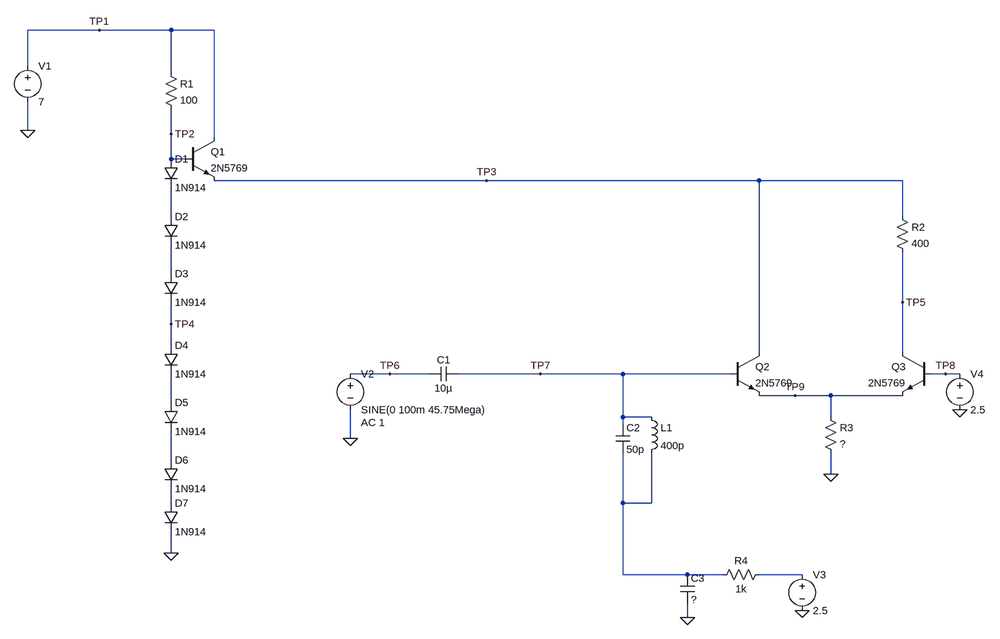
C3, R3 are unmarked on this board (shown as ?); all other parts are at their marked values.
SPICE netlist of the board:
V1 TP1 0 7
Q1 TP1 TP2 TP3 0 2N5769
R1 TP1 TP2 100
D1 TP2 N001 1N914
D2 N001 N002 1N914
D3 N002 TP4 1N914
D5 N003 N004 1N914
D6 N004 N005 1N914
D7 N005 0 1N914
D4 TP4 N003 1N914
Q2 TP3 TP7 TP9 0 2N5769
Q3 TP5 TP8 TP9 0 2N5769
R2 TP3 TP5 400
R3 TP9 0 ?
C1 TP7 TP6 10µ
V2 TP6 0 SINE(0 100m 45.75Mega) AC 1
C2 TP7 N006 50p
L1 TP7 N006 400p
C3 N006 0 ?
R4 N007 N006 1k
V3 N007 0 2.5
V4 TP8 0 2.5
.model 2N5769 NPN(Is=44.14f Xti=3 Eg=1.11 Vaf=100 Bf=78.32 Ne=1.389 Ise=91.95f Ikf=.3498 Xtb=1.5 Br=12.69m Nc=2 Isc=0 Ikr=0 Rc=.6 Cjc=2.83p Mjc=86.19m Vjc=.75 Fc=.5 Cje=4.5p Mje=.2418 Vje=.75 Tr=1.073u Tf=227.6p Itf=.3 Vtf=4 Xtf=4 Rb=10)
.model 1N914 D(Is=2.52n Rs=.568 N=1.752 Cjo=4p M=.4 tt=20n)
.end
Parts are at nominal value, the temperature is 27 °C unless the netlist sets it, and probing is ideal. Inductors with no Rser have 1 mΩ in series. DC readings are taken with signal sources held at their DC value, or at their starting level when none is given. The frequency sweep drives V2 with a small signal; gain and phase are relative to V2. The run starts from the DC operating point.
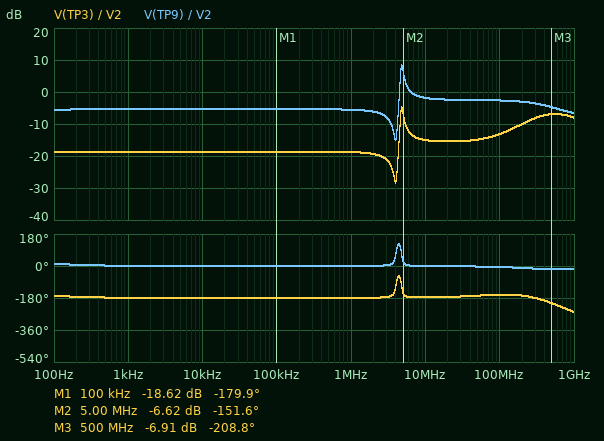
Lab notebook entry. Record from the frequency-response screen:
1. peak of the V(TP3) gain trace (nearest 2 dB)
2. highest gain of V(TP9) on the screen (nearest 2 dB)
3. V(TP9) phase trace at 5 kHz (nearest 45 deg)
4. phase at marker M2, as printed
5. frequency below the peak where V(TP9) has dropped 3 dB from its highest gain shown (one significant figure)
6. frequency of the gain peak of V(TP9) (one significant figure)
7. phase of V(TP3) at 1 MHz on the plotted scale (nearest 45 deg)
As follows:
-4 dB
8 dB
0 deg
-151.6 deg
5 MHz
5 MHz
-180 deg
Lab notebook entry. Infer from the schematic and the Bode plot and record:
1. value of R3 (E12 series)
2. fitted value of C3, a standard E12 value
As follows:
68 Ω
3.9 µF
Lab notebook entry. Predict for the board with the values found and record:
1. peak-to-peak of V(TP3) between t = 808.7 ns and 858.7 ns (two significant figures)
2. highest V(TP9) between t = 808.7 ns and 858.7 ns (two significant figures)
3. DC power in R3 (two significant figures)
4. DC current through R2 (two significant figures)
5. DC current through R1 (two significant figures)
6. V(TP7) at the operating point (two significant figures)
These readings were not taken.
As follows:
34 mV
1.8 V
43 mW
6.4 mA
19 mA
2.4 V
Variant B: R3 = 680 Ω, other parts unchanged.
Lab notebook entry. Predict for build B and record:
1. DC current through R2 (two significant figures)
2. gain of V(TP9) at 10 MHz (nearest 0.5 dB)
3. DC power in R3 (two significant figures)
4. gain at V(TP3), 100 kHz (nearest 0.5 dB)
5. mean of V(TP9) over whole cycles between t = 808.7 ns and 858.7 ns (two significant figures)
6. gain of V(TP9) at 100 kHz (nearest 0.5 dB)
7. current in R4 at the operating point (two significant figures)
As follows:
1.7 mA
-8.0 dB
5.1 mW
-48.5 dB
1.9 V
-11.5 dB
15 µA
